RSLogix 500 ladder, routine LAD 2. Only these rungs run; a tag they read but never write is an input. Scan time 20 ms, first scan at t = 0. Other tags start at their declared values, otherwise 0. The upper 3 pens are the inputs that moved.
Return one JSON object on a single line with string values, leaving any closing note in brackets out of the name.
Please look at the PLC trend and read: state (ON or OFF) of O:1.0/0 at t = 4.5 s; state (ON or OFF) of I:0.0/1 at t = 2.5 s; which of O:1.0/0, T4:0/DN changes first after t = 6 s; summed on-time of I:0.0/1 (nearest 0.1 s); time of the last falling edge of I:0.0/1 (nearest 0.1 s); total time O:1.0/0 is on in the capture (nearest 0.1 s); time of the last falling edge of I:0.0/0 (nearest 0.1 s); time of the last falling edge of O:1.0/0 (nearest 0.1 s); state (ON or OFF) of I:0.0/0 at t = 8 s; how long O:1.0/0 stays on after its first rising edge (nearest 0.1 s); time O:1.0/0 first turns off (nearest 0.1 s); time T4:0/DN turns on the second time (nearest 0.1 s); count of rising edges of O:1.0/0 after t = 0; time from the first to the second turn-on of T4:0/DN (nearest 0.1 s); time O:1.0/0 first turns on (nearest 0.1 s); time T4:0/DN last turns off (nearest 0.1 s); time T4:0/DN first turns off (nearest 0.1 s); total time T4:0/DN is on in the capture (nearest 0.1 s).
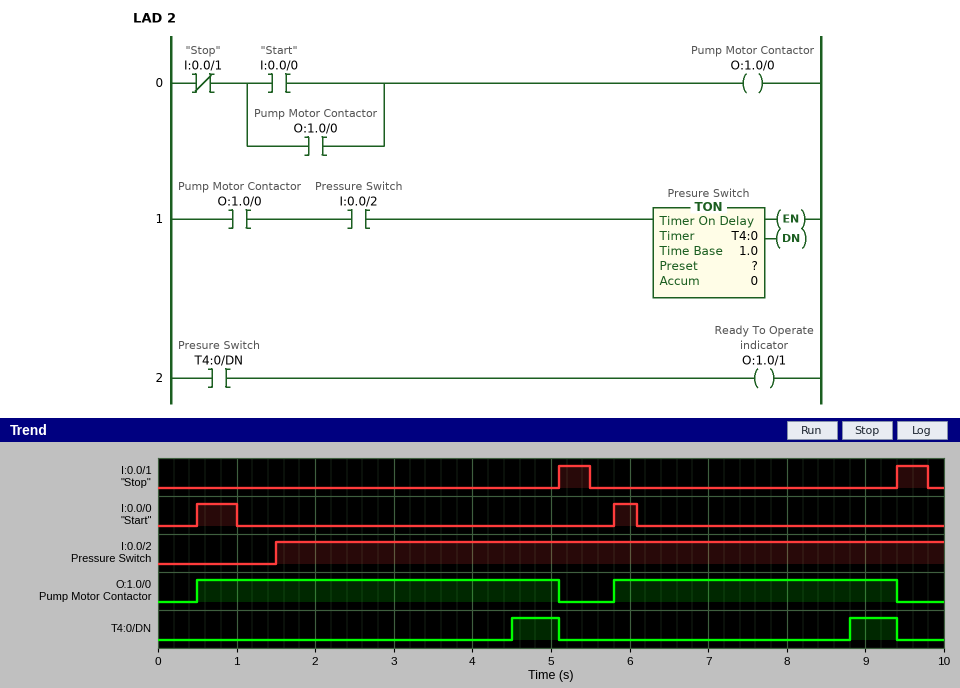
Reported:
{"state (ON or OFF) of O:1.0/0 at t = 4.5 s": "ON", "state (ON or OFF) of I:0.0/1 at t = 2.5 s": "OFF", "which of O:1.0/0, T4:0/DN changes first after t = 6 s": "T4:0/DN", "summed on-time of I:0.0/1": "0.8 s", "time of the last falling edge of I:0.0/1": "9.8 s", "total time O:1.0/0 is on in the capture": "8.2 s", "time of the last falling edge of I:0.0/0": "6.1 s", "time of the last falling edge of O:1.0/0": "9.4 s", "state (ON or OFF) of I:0.0/0 at t = 8 s": "OFF", "how long O:1.0/0 stays on after its first rising edge": "4.6 s", "time O:1.0/0 first turns off": "5.1 s", "time T4:0/DN turns on the second time": "8.8 s", "count of rising edges of O:1.0/0 after t = 0": "2", "time from the first to the second turn-on of T4:0/DN": "4.3 s", "time O:1.0/0 first turns on": "0.5 s", "time T4:0/DN last turns off": "9.4 s", "time T4:0/DN first turns off": "5.1 s", "total time T4:0/DN is on in the capture": "1.2 s"}
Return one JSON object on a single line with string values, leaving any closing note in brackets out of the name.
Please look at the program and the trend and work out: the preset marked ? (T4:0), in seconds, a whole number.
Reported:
{"the preset marked ? (T4:0), in seconds, a whole number": "3 s"}
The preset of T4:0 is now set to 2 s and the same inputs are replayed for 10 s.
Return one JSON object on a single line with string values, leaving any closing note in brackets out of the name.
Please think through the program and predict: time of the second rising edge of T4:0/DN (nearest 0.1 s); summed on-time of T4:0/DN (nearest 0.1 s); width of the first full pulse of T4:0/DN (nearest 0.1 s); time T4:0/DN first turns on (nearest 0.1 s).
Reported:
{"time of the second rising edge of T4:0/DN": "7.8 s", "summed on-time of T4:0/DN": "3.2 s", "width of the first full pulse of T4:0/DN": "1.6 s", "time T4:0/DN first turns on": "3.5 s"}
